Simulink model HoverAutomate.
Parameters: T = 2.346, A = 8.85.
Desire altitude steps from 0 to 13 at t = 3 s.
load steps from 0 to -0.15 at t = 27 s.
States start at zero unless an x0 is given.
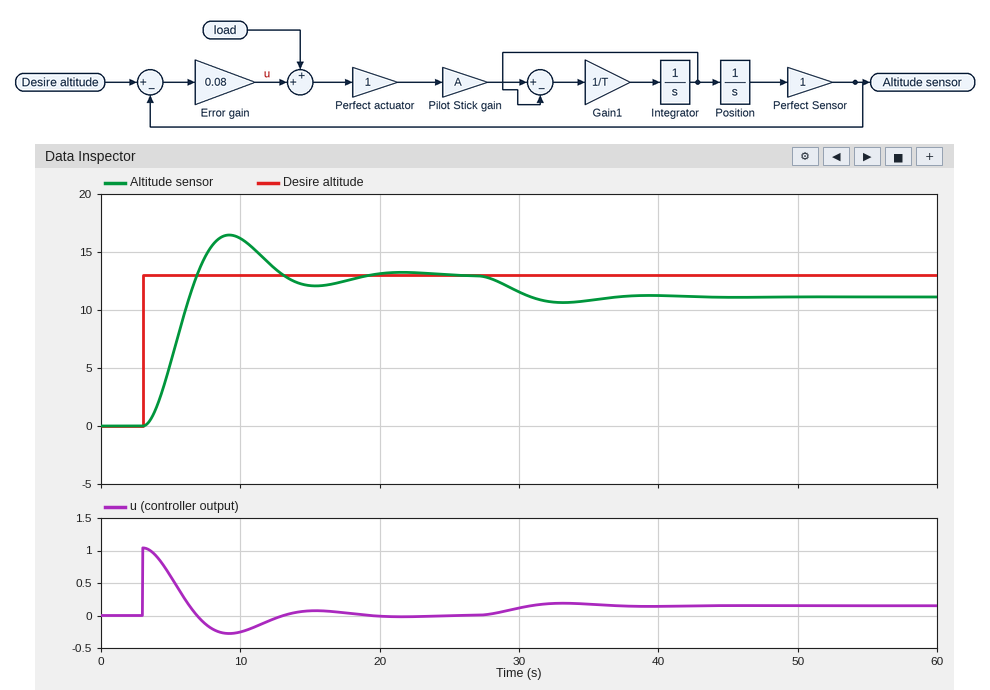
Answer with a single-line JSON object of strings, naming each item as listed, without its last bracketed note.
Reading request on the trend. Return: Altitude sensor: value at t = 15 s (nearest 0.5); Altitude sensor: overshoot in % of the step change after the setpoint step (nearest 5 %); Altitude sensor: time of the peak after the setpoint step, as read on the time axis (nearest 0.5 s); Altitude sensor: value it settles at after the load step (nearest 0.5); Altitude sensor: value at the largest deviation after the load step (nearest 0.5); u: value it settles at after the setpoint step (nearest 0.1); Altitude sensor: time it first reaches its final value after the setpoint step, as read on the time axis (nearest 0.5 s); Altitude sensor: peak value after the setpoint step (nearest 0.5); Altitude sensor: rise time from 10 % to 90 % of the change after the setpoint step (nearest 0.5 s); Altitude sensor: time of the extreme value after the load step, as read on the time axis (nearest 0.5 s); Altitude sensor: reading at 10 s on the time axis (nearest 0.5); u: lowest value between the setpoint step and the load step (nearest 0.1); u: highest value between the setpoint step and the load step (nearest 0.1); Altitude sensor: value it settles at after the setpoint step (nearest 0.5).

{"Altitude sensor: value at t = 15 s": "12.0", "Altitude sensor: overshoot in % of the step change after the setpoint step": "25 %", "Altitude sensor: time of the peak after the setpoint step, as read on the time axis": "9.0 s", "Altitude sensor: value it settles at after the load step": "11.0", "Altitude sensor: value at the largest deviation after the load step": "10.5", "u: value it settles at after the setpoint step": "0.0", "Altitude sensor: time it first reaches its final value after the setpoint step, as read on the time axis": "7.0 s", "Altitude sensor: peak value after the setpoint step": "16.5", "Altitude sensor: rise time from 10 % to 90 % of the change after the setpoint step": "2.5 s", "Altitude sensor: time of the extreme value after the load step, as read on the time axis": "33.0 s", "Altitude sensor: reading at 10 s on the time axis": "16.0", "u: lowest value between the setpoint step and the load step": "-0.3", "u: highest value between the setpoint step and the load step": "1.0", "Altitude sensor: value it settles at after the setpoint step": "13.0"}
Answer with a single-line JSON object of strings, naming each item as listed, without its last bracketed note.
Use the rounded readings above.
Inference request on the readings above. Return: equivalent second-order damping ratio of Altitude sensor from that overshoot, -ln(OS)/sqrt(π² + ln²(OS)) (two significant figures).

{"equivalent second-order damping ratio of Altitude sensor from that overshoot, -ln(OS)/sqrt(π² + ln²(OS))": "0.40"}
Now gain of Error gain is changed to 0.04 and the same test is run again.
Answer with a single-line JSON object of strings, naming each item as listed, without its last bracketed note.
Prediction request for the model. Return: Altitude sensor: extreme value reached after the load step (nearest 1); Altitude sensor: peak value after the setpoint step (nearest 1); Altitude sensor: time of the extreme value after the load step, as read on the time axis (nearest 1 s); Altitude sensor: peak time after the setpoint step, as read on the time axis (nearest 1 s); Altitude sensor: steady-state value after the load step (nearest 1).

{"Altitude sensor: extreme value reached after the load step": "9", "Altitude sensor: peak value after the setpoint step": "15", "Altitude sensor: time of the extreme value after the load step, as read on the time axis": "37 s", "Altitude sensor: peak time after the setpoint step, as read on the time axis": "13 s", "Altitude sensor: steady-state value after the load step": "9"}
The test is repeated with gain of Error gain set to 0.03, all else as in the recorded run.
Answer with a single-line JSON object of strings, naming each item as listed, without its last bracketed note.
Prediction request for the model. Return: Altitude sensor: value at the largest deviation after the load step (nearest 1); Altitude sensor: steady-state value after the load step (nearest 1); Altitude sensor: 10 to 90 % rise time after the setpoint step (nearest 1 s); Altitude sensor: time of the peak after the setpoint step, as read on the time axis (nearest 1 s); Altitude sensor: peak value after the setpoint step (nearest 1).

{"Altitude sensor: value at the largest deviation after the load step": "8", "Altitude sensor: steady-state value after the load step": "8", "Altitude sensor: 10 to 90 % rise time after the setpoint step": "6 s", "Altitude sensor: time of the peak after the setpoint step, as read on the time axis": "15 s", "Altitude sensor: peak value after the setpoint step": "14"}
